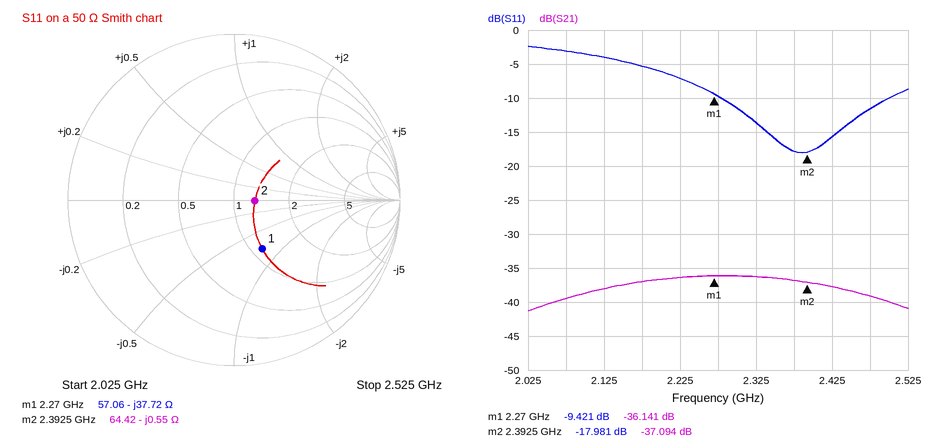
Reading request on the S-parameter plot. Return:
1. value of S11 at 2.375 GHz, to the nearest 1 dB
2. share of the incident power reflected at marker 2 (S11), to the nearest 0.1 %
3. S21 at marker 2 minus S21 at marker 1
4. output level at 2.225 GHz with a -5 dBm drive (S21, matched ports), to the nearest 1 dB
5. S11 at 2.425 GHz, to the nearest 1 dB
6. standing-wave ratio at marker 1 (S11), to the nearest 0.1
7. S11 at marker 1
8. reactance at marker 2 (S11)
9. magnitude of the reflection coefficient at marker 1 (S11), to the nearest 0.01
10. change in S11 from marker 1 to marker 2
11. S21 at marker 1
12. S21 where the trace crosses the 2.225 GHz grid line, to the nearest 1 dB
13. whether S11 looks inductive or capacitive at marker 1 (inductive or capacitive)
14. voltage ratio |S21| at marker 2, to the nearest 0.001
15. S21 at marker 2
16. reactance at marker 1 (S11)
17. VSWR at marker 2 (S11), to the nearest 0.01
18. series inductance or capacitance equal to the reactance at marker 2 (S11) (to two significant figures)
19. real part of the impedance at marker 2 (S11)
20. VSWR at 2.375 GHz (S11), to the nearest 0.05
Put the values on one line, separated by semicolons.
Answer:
-18 dB; 1.6 %; -0.953 dB; -41 dBm; -16 dB; 2.0; -9.421 dB; -0.55 Ω; 0.34; -8.560 dB; -36.141 dB; -36 dB; capacitive; 0.014; -37.094 dB; -37.72 Ω; 1.29; 120 pF; 64.42 Ω; 1.30
